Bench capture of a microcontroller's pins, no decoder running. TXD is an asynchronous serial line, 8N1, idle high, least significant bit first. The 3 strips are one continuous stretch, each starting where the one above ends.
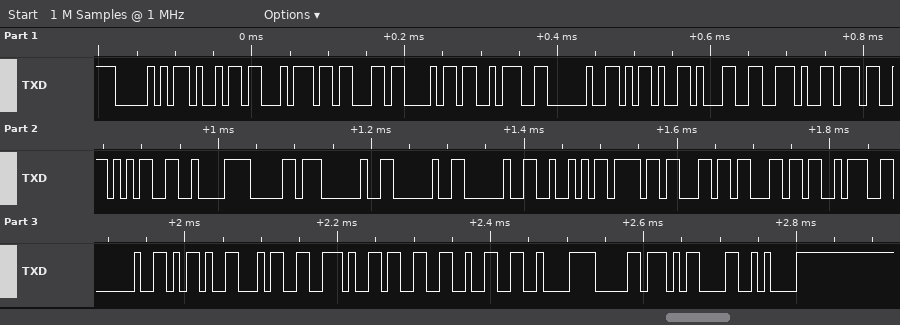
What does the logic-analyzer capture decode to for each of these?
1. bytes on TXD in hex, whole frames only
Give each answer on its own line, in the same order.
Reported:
0x50 0x69 0x74 0x63 0x68 0x3A 0x20 0x2D 0x31 0x2E 0x37 0x35 0xC2 0xB0 0x20 0x20 0x20 0x52 0x6F 0x6C 0x6C 0x3A 0x20 0x2D 0x34 0x2E 0x33 0x32 0xC2 0xB0 0x0D 0x0A
